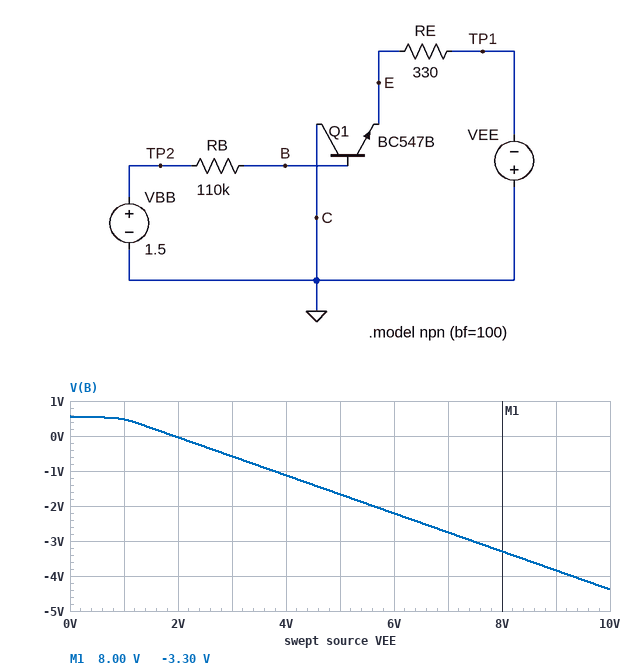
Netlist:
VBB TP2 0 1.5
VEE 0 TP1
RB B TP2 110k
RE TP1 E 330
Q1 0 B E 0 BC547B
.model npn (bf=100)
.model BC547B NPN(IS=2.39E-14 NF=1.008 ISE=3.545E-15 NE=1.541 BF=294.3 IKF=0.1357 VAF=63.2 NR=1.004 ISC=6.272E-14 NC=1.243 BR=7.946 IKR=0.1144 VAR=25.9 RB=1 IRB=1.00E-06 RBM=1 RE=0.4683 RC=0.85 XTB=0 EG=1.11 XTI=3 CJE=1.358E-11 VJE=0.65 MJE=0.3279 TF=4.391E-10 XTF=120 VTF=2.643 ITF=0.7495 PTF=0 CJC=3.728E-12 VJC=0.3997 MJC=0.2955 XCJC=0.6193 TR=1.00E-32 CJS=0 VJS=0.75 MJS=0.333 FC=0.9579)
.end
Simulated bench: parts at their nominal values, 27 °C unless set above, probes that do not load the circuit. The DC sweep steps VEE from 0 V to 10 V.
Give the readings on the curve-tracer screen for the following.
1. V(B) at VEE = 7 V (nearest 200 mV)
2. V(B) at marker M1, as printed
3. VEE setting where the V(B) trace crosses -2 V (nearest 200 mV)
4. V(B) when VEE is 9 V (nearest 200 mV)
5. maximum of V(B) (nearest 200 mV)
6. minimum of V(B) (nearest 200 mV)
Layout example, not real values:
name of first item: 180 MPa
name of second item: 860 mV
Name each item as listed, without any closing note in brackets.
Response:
V(B) at VEE = 7 V: -2.8 V
V(B) at marker M1, as printed: -3.30 V
VEE setting where the V(B) trace crosses -2 V: 5.6 V
V(B) when VEE is 9 V: -3.8 V
maximum of V(B): 600 mV
minimum of V(B): -4.4 V
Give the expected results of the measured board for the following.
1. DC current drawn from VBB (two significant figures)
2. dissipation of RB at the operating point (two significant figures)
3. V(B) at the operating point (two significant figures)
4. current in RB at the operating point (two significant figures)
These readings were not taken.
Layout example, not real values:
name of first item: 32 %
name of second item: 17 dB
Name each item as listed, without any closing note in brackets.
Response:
DC current drawn from VBB: 8.6 µA
dissipation of RB at the operating point: 8.1 µW
V(B) at the operating point: 560 mV
current in RB at the operating point: 8.6 µA
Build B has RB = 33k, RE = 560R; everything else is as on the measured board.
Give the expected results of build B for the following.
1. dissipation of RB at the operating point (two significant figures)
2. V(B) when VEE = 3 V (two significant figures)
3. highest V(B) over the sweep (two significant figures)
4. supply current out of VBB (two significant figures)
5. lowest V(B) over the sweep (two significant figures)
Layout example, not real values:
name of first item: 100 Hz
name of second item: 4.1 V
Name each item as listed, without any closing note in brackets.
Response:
dissipation of RB at the operating point: 25 µW
V(B) when VEE = 3 V: 560 mV
highest V(B) over the sweep: 590 mV
supply current out of VBB: 28 µA
lowest V(B) over the sweep: -500 mV
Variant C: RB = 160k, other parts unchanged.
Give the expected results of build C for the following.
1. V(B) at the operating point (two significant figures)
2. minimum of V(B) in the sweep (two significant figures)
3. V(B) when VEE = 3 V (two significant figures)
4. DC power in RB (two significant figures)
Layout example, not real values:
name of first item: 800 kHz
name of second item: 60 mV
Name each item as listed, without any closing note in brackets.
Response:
V(B) at the operating point: 550 mV
minimum of V(B) in the sweep: -5.3 V
V(B) when VEE = 3 V: -920 mV
DC power in RB: 5.7 µW
